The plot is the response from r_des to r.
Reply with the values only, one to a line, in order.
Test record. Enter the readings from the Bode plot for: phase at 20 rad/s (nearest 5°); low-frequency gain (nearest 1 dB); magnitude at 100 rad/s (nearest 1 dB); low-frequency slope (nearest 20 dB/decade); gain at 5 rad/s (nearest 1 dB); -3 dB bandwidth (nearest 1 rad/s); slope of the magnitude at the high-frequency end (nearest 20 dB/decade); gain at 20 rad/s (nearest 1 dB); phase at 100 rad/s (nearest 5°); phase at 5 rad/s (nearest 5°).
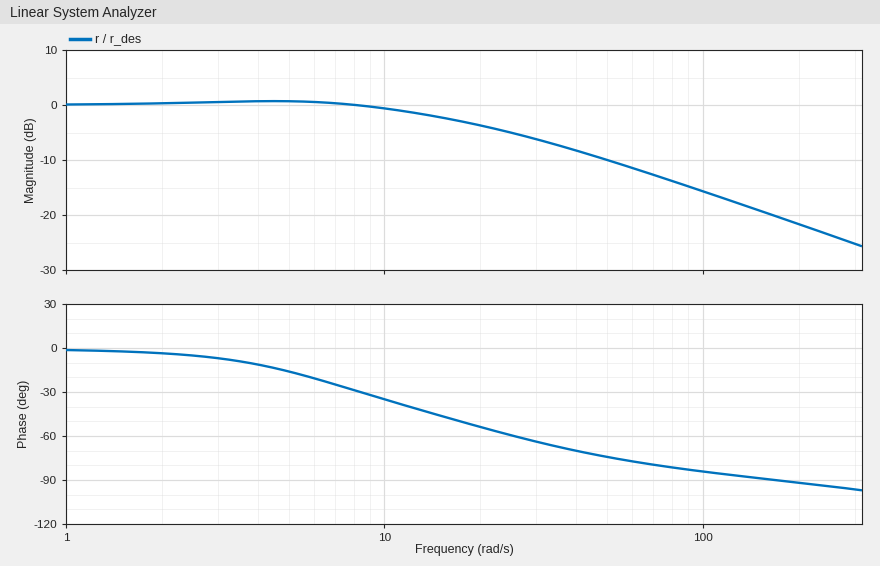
-55°
0 dB
-16 dB
0 dB/decade
1 dB
17 rad/s
-20 dB/decade
-4 dB
-85°
-15°
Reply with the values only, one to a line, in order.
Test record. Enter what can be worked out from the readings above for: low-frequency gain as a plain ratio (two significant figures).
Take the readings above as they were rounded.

1.0
